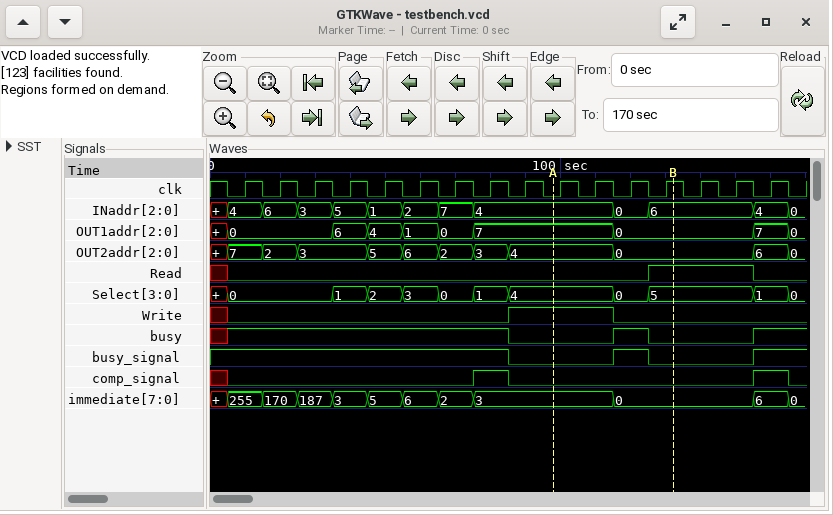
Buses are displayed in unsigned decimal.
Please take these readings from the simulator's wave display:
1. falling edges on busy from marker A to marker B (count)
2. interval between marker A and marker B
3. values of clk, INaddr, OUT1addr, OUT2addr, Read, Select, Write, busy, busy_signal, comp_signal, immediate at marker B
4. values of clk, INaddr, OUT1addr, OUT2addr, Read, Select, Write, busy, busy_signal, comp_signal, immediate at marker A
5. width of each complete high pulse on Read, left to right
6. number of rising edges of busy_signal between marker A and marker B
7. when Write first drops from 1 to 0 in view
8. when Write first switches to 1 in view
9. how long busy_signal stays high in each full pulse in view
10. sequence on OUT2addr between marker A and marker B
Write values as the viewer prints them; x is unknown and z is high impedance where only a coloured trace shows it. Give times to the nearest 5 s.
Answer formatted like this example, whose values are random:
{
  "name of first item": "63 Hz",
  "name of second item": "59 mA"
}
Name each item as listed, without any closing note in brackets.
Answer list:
{
  "falling edges on busy from marker A to marker B": "1",
  "interval between marker A and marker B": "35 s",
  "values of clk, INaddr, OUT1addr, OUT2addr, Read, Select, Write, busy, busy_signal, comp_signal, immediate at marker B": "clk=1, INaddr=6, OUT1addr=0, OUT2addr=0, Read=1, Select=5, Write=0, busy=0, busy_signal=0, comp_signal=0, immediate=0",
  "values of clk, INaddr, OUT1addr, OUT2addr, Read, Select, Write, busy, busy_signal, comp_signal, immediate at marker A": "clk=0, INaddr=4, OUT1addr=7, OUT2addr=4, Read=0, Select=4, Write=1, busy=0, busy_signal=0, comp_signal=0, immediate=3",
  "width of each complete high pulse on Read, left to right": "30 s",
  "number of rising edges of busy_signal between marker A and marker B": "1",
  "when Write first drops from 1 to 0 in view": "115 s",
  "when Write first switches to 1 in view": "85 s",
  "how long busy_signal stays high in each full pulse in view": "10 s",
  "sequence on OUT2addr between marker A and marker B": "4, 0"
}
